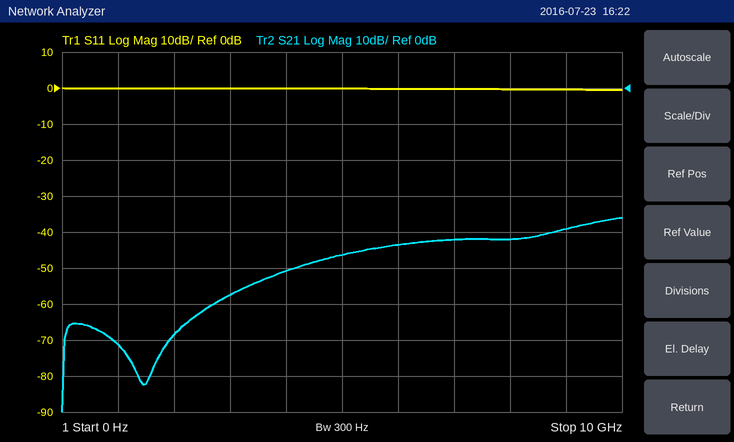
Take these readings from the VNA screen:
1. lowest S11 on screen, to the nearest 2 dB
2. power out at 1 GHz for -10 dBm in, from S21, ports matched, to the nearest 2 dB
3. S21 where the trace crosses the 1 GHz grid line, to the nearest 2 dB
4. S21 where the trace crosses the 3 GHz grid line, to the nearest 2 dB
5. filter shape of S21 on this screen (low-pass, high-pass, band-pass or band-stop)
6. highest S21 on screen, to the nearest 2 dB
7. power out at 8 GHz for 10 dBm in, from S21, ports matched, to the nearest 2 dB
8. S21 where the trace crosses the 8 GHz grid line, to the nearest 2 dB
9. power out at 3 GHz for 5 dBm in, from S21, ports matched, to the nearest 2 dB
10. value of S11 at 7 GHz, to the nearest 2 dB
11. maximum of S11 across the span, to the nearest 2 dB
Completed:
0 dB
-82 dBm
-72 dB
-58 dB
high-pass
-36 dB
-32 dBm
-42 dB
-52 dBm
0 dB
0 dB
